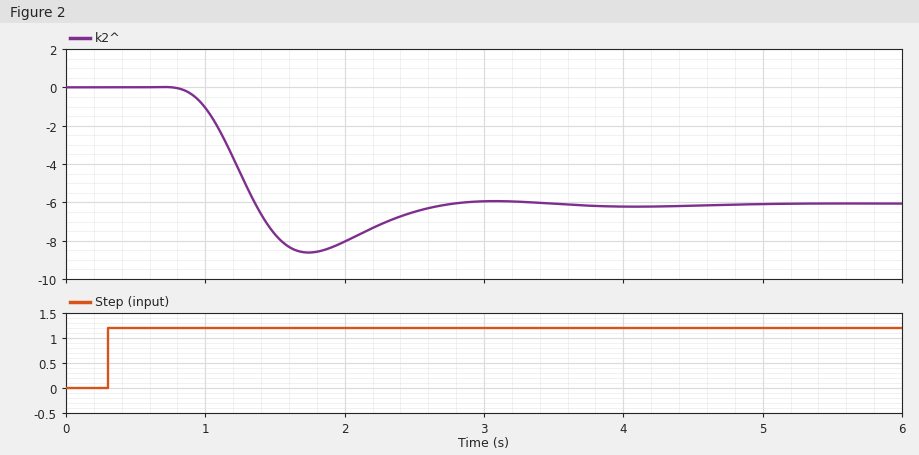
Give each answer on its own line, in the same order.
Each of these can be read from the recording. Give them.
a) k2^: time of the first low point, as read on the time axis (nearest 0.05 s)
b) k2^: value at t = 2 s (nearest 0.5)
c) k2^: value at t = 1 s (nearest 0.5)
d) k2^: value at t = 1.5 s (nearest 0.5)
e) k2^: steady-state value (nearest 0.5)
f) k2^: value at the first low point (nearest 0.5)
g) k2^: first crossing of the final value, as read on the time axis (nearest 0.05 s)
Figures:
1.75 s
-8.0
-1.0
-7.5
-6.0
-8.5
1.35 s
